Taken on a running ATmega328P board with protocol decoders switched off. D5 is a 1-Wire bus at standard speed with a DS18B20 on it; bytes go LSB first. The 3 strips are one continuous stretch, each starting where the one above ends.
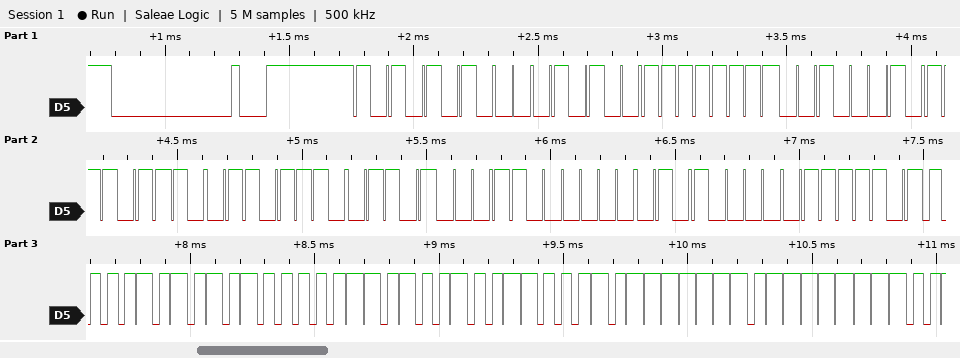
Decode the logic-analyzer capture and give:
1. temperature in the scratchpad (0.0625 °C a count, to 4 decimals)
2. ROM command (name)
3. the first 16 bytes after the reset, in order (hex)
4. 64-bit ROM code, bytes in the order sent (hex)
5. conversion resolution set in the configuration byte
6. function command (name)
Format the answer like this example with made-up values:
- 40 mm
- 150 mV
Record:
- 85.0000 °C
- Match ROM
- 55 28 FF 44 77 76 16 03 0A BE 50 05 4B 46 7F FF
- 28 FF 44 77 76 16 03 0A
- 12 bits
- Read Scratchpad
